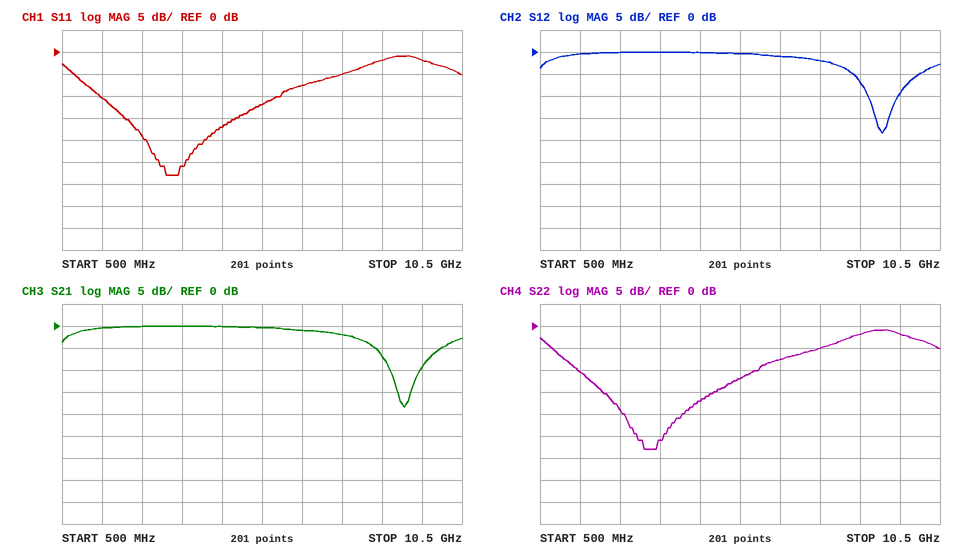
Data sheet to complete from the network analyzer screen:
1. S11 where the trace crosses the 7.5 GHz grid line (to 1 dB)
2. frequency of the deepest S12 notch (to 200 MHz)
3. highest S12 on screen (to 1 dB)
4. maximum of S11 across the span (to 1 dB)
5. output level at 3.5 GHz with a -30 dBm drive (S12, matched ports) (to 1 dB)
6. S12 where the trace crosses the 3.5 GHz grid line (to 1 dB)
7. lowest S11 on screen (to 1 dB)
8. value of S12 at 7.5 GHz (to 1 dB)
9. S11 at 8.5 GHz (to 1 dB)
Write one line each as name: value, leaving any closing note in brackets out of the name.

S11 where the trace crosses the 7.5 GHz grid line: -5 dB
frequency of the deepest S12 notch: 9.0 GHz
highest S12 on screen: 0 dB
maximum of S11 across the span: -1 dB
output level at 3.5 GHz with a -30 dBm drive (S12, matched ports): -30 dBm
S12 where the trace crosses the 3.5 GHz grid line: 0 dB
lowest S11 on screen: -28 dB
value of S12 at 7.5 GHz: -2 dB
S11 at 8.5 GHz: -2 dB
